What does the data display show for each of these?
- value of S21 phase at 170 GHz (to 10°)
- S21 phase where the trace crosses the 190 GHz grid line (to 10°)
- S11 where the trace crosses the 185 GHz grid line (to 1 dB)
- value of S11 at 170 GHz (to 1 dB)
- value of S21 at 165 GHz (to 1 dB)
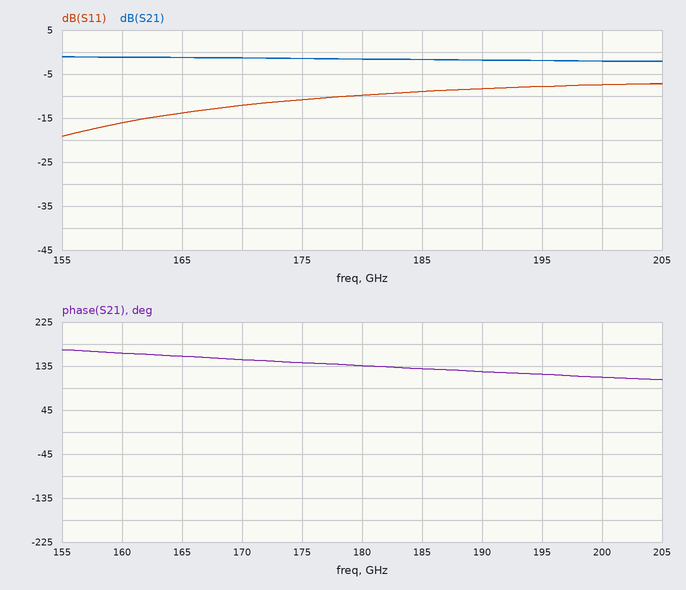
150°
120°
-9 dB
-12 dB
-1 dB
